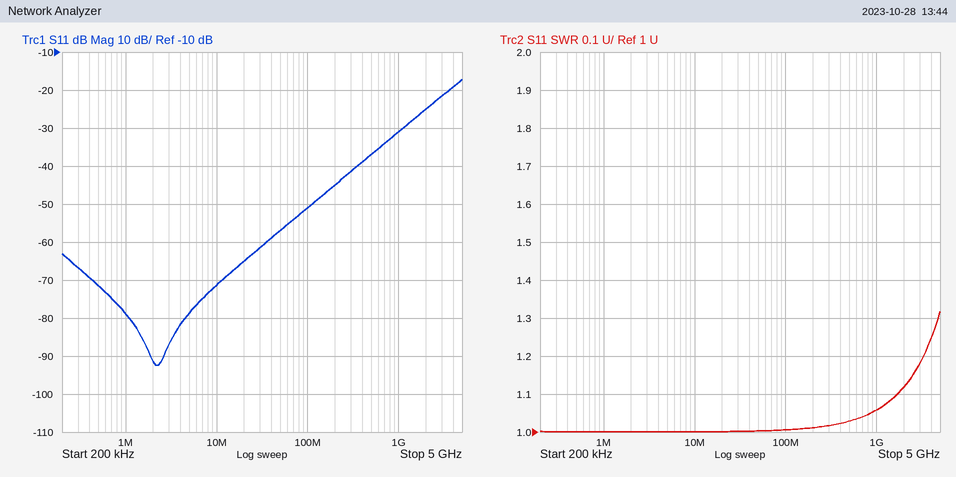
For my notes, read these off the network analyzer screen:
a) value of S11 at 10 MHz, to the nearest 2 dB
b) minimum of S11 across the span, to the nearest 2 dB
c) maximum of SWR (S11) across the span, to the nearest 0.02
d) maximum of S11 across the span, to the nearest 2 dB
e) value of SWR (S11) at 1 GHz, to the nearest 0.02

-72 dB
-92 dB
1.32
-18 dB
1.06
